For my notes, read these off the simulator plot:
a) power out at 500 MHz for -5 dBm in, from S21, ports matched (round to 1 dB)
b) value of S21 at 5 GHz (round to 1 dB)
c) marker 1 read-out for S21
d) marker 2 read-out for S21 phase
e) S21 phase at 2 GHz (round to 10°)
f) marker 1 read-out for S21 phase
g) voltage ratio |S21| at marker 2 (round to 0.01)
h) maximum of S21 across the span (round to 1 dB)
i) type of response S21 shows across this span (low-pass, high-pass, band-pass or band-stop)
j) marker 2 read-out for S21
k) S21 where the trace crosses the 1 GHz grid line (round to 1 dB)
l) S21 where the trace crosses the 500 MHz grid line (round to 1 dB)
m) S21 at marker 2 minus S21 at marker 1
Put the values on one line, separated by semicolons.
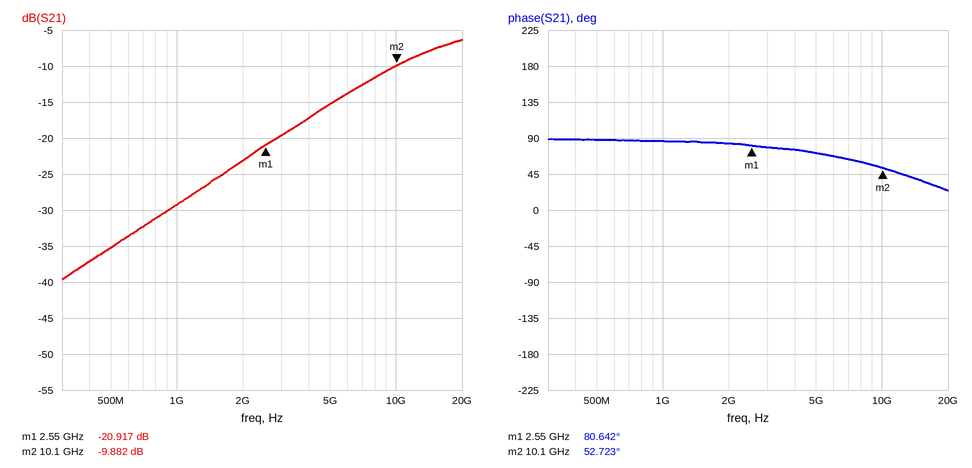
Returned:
-40 dBm; -15 dB; -20.917 dB; 52.723°; 80°; 80.642°; 0.32; -6 dB; high-pass; -9.882 dB; -29 dB; -35 dB; 11.035 dB
